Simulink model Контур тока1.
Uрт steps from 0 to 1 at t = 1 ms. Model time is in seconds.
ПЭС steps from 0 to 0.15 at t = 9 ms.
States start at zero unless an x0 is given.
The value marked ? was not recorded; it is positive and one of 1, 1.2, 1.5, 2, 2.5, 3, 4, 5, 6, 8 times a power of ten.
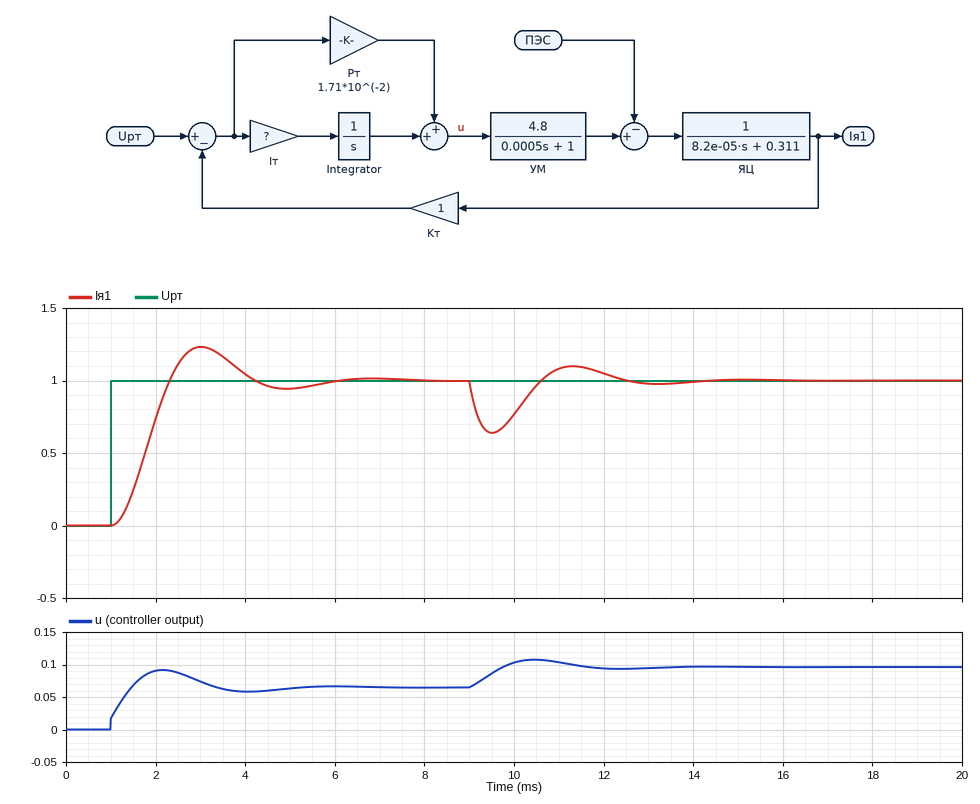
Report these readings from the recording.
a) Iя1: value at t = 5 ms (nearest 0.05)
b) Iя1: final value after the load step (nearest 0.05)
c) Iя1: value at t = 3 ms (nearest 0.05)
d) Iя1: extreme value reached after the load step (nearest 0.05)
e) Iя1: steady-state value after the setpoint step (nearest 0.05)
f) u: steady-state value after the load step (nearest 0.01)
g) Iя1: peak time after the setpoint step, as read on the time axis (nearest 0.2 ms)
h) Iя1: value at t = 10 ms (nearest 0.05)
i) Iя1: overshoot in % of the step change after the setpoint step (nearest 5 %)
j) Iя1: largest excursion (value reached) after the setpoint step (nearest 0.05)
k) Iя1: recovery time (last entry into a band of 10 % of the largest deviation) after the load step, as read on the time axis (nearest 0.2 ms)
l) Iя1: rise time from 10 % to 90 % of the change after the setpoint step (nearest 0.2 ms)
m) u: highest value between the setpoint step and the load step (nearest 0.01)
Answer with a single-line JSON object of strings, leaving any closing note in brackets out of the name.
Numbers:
{"Iя1: value at t = 5 ms": "0.95", "Iя1: final value after the load step": "1.00", "Iя1: value at t = 3 ms": "1.25", "Iя1: extreme value reached after the load step": "0.65", "Iя1: steady-state value after the setpoint step": "1.00", "u: steady-state value after the load step": "0.10", "Iя1: peak time after the setpoint step, as read on the time axis": "3.0 ms", "Iя1: value at t = 10 ms": "0.75", "Iя1: overshoot in % of the step change after the setpoint step": "25 %", "Iя1: largest excursion (value reached) after the setpoint step": "1.25", "Iя1: recovery time (last entry into a band of 10 % of the largest deviation) after the load step, as read on the time axis": "12.2 ms", "Iя1: rise time from 10 % to 90 % of the change after the setpoint step": "0.8 ms", "u: highest value between the setpoint step and the load step": "0.09"}
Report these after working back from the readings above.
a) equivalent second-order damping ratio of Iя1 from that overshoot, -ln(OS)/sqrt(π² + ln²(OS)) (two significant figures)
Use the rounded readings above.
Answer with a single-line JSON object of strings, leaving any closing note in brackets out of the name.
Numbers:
{"equivalent second-order damping ratio of Iя1 from that overshoot, -ln(OS)/sqrt(π² + ln²(OS))": "0.40"}
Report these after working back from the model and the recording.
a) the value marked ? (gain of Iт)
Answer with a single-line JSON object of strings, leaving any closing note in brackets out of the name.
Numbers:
{"the value marked ?": "120"}
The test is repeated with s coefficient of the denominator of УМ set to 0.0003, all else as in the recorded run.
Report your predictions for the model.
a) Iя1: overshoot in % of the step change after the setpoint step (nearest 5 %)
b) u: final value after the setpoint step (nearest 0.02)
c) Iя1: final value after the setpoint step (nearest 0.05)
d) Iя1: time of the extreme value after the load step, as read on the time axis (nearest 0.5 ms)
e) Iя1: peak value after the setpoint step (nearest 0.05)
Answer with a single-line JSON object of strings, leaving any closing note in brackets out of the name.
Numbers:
{"Iя1: overshoot in % of the step change after the setpoint step": "15 %", "u: final value after the setpoint step": "0.06", "Iя1: final value after the setpoint step": "1.00", "Iя1: time of the extreme value after the load step, as read on the time axis": "9.5 ms", "Iя1: peak value after the setpoint step": "1.15"}
